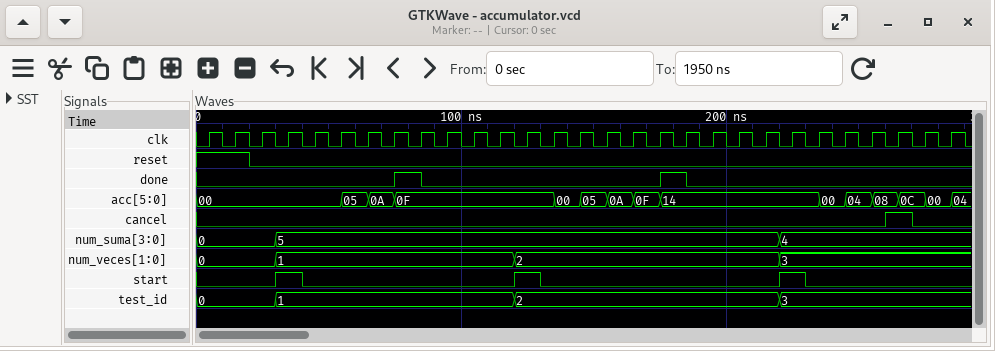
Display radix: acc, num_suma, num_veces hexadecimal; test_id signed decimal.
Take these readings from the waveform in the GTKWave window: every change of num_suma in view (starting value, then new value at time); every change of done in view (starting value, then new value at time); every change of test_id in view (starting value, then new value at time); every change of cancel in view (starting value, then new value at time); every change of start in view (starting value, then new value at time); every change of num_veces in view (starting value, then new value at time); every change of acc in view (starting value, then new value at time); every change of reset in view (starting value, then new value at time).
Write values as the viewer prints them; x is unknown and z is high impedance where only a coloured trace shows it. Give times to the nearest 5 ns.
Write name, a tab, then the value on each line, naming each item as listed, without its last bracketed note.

every change of num_suma in view	0, 5 at 30 ns, 4 at 220 ns
every change of done in view	0, 1 at 75 ns, 0 at 85 ns, 1 at 175 ns, 0 at 185 ns
every change of test_id in view	0, 1 at 30 ns, 2 at 120 ns, 3 at 220 ns
every change of cancel in view	0, 1 at 260 ns, 0 at 270 ns
every change of start in view	0, 1 at 30 ns, 0 at 40 ns, 1 at 120 ns, 0 at 130 ns, 1 at 220 ns, 0 at 230 ns
every change of num_veces in view	0, 1 at 30 ns, 2 at 120 ns, 3 at 220 ns
every change of acc in view	00, 05 at 55 ns, 0A at 65 ns, 0F at 75 ns, 00 at 135 ns, 05 at 145 ns, 0A at 155 ns, 0F at 165 ns, 14 at 175 ns, 00 at 235 ns, 04 at 245 ns, 08 at 255 ns, 0C at 265 ns, 00 at 275 ns, 04 at 285 ns
every change of reset in view	1, 0 at 20 ns
